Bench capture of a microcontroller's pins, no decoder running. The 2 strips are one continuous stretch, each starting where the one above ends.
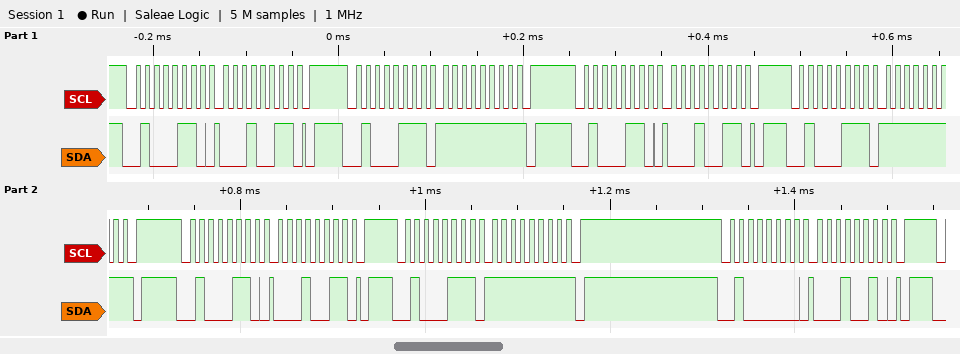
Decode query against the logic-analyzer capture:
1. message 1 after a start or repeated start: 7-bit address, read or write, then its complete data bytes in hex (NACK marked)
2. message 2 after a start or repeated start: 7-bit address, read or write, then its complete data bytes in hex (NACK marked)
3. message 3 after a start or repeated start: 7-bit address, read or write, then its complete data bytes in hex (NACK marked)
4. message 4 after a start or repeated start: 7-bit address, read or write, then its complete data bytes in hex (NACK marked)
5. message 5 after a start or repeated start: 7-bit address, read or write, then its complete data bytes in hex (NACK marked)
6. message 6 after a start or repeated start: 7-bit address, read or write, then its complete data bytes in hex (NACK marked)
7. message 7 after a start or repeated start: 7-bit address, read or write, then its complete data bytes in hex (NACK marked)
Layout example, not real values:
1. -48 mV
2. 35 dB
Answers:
1. 0x23 write: 13
2. 0x23 read: FF NACK
3. 0x23 write: 13
4. 0x23 read: FF NACK
5. 0x23 write: 13
6. 0x23 read: FF NACK
7. 0x20 write: 12
